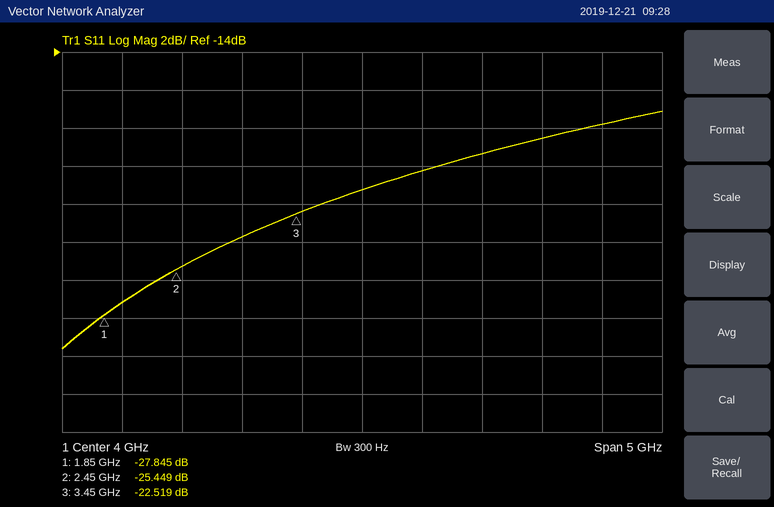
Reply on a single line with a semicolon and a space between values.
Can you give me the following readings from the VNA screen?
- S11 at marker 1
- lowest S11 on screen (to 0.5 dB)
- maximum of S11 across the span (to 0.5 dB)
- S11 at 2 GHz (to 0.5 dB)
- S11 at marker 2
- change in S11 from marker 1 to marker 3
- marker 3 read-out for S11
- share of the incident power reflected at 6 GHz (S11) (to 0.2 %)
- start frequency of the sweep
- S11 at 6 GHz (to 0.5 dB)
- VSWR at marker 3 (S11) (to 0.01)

-27.845 dB; -29.5 dB; -17.0 dB; -27.0 dB; -25.449 dB; 5.326 dB; -22.519 dB; 1.6 %; 1.5 GHz; -18.0 dB; 1.16
